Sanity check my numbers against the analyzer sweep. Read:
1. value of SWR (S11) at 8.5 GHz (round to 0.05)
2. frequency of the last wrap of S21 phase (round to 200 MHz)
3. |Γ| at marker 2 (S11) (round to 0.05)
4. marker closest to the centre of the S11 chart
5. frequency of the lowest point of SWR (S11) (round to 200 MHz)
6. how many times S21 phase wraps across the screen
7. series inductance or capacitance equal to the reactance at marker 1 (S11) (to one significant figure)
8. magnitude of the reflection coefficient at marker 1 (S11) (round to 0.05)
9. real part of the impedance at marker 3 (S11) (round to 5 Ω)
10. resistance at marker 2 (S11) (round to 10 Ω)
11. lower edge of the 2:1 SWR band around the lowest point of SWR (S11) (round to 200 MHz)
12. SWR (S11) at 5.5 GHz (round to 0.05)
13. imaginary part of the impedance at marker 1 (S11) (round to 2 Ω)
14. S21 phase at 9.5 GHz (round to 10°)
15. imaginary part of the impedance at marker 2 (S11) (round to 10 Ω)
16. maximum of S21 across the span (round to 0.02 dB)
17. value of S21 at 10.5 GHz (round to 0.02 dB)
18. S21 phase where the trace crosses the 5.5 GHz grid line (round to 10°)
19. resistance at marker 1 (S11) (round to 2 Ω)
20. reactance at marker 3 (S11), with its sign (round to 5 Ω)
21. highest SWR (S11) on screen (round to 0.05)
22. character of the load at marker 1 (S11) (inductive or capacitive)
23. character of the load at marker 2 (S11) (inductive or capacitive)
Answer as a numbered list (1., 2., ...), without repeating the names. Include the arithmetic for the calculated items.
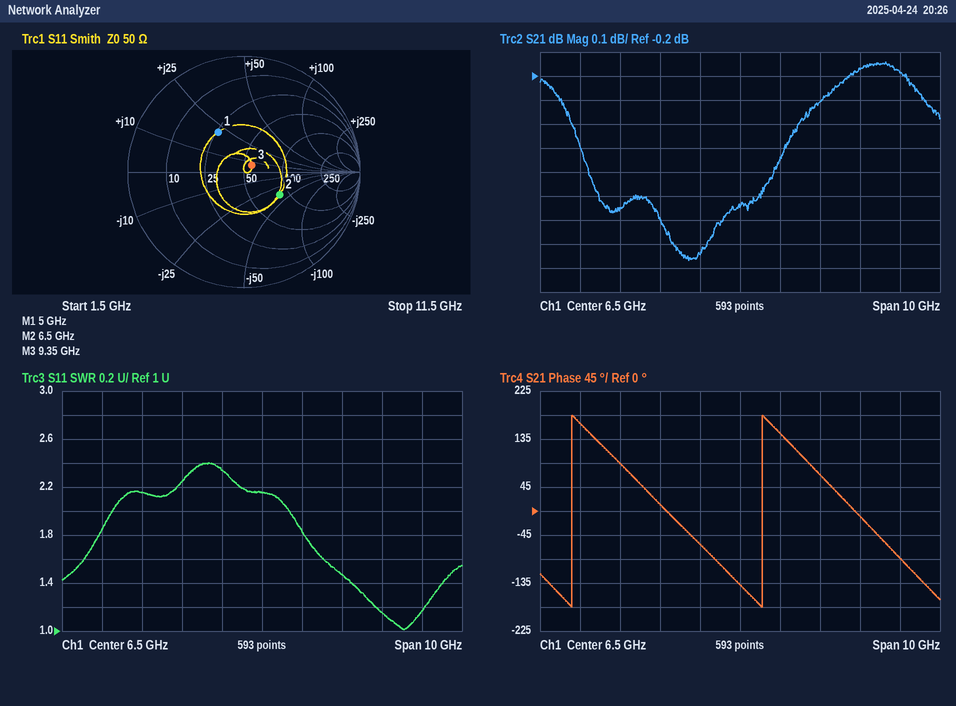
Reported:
1. 1.45
2. 7.0 GHz
3. 0.35
4. marker 3
5. 10.0 GHz
6. 2
7. L = 22 Ω/(2π × 5 GHz) ≈ 700 pH
8. 0.40
9. 55 Ω
10. 80 Ω
11. 7.2 GHz
12. 2.35
13. +22 Ω
14. -10°
15. -40 Ω
16. -0.14 dB
17. -0.18 dB
18. -60°
19. 26 Ω
20. +5 Ω
21. 2.40
22. inductive
23. capacitive
